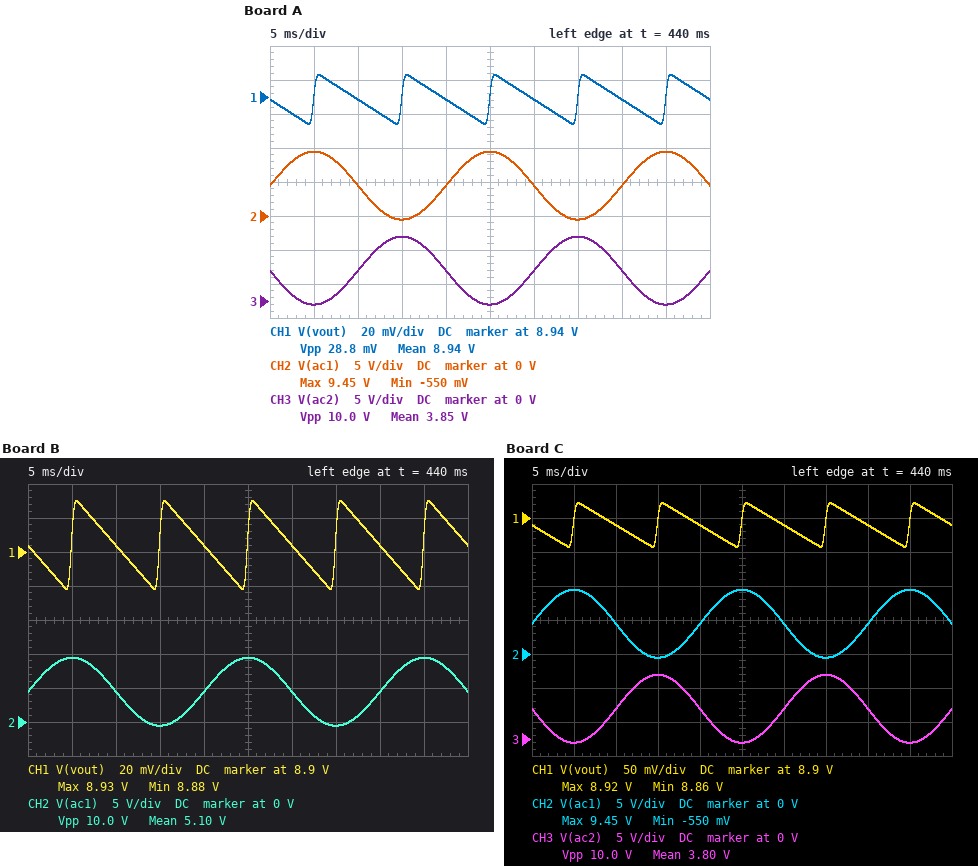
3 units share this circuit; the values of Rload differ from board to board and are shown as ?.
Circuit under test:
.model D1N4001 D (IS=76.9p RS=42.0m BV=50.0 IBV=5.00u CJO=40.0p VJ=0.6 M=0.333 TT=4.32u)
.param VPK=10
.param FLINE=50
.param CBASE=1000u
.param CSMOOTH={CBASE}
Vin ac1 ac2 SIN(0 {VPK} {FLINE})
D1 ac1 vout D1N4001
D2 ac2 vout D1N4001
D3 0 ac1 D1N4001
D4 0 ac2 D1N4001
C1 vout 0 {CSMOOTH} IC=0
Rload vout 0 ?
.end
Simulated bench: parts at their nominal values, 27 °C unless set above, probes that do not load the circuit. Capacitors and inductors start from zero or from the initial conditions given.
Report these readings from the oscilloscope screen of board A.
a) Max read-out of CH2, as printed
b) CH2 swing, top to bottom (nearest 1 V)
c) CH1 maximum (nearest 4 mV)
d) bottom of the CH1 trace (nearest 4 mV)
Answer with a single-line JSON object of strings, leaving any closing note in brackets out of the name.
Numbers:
{"Max read-out of CH2, as printed": "9.45 V", "CH2 swing, top to bottom": "10 V", "CH1 maximum": "8.952 V", "bottom of the CH1 trace": "8.924 V"}
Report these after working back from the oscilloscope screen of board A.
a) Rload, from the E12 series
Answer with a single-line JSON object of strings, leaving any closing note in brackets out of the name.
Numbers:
{"Rload, from the E12 series": "2.7 kΩ"}
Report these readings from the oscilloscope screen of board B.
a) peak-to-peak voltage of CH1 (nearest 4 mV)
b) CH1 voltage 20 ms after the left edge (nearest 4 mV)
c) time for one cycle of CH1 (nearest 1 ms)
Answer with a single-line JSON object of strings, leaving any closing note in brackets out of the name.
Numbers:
{"peak-to-peak voltage of CH1": "52 mV", "CH1 voltage 20 ms after the left edge": "8.904 V", "time for one cycle of CH1": "10 ms"}
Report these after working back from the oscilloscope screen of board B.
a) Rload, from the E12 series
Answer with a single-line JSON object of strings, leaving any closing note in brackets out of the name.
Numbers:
{"Rload, from the E12 series": "1.5 kΩ"}
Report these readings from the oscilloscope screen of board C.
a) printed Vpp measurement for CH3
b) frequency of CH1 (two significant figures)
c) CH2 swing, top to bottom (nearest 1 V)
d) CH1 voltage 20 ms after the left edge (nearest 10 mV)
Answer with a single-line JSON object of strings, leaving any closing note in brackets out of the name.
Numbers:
{"printed Vpp measurement for CH3": "10.0 V", "frequency of CH1": "100 Hz", "CH2 swing, top to bottom": "10 V", "CH1 voltage 20 ms after the left edge": "8.89 V"}
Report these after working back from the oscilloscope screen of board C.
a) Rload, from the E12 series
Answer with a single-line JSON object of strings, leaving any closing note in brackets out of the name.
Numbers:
{"Rload, from the E12 series": "1.2 kΩ"}
